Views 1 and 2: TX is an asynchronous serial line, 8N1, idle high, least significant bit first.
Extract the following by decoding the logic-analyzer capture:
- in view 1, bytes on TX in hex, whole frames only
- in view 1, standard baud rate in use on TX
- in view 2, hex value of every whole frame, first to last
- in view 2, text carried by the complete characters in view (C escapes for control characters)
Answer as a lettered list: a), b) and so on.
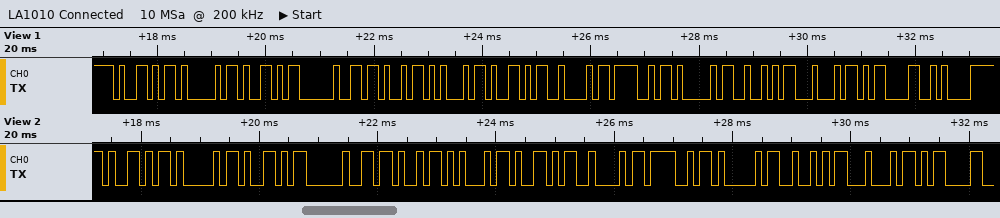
a) 59 41 59 20 4B 45 59 42 4F 41 52 44 0D 0A
b) 9600 baud
c) 59 41 59 20 4B 45 59 42 4F 41 52 44 0D
d) "YAY KEYBOARD\r"
